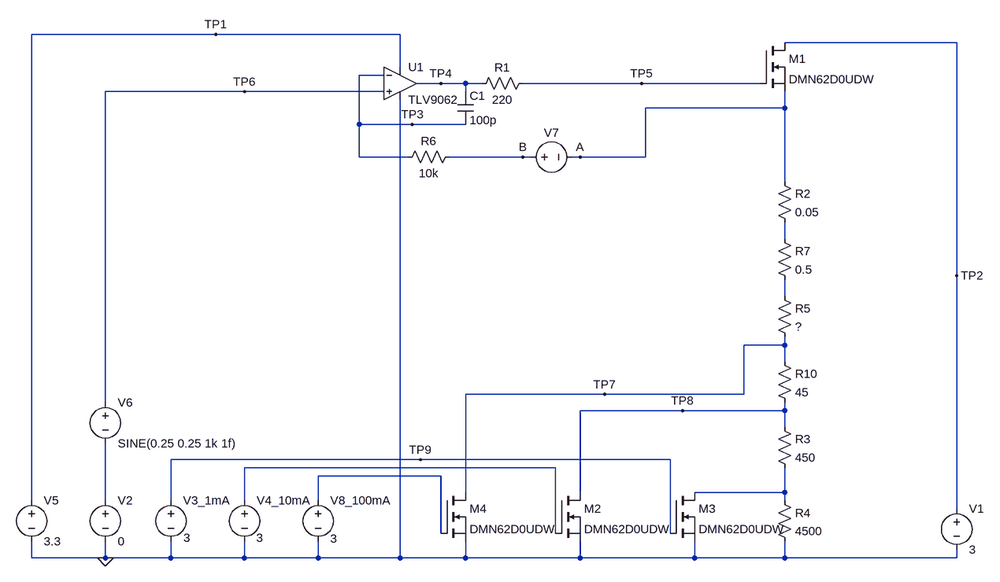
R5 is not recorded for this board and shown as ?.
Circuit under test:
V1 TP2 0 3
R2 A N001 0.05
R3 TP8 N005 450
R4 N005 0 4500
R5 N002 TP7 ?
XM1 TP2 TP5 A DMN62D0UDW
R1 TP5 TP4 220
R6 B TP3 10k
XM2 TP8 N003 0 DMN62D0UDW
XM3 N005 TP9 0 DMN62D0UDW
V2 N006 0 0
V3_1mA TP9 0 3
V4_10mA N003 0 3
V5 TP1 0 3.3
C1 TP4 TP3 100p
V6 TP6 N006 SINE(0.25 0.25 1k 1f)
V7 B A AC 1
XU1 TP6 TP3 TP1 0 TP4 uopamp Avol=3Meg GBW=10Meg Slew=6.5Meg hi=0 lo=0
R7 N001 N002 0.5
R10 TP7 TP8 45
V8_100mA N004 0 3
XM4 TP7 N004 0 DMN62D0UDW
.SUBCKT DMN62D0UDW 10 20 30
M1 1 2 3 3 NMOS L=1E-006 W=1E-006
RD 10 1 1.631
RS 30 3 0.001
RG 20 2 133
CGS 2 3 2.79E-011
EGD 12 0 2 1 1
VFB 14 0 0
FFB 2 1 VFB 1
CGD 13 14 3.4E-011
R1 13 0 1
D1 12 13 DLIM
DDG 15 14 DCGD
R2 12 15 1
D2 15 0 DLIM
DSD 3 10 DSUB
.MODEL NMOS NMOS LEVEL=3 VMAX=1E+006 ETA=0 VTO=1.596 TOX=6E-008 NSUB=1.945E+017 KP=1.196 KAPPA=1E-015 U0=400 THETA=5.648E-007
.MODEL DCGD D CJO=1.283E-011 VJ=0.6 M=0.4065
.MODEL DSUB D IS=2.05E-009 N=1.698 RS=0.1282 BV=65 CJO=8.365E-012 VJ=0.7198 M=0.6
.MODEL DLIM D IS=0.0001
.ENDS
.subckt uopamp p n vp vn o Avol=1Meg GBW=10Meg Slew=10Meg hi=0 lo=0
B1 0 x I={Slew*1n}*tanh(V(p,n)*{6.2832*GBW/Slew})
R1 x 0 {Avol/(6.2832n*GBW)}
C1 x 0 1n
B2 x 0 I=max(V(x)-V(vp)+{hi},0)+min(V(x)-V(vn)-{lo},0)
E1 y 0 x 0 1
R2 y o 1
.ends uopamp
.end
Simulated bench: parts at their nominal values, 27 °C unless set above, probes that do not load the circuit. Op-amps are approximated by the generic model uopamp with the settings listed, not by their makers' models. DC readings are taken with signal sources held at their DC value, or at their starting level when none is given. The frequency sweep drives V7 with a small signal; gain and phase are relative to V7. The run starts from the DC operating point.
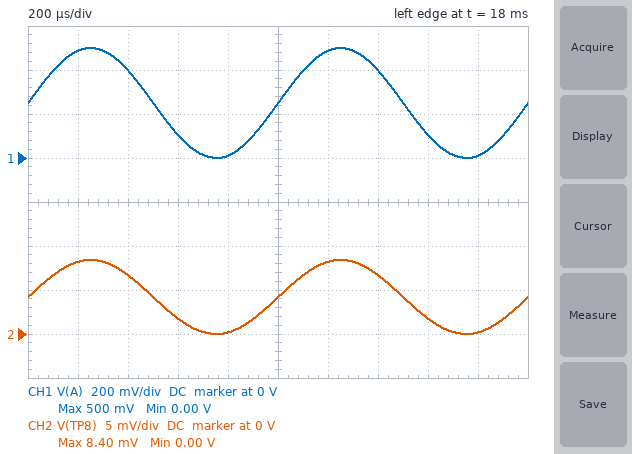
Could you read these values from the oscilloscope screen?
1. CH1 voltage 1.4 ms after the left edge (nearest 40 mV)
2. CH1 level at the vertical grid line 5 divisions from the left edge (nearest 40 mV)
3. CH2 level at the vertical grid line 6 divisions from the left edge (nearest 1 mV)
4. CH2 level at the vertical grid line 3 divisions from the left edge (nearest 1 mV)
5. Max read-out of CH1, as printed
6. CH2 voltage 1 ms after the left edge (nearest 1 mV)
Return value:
400 mV
240 mV
8 mV
2 mV
500 mV
4 mV
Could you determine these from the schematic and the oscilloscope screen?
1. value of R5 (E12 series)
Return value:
3.3 Ω
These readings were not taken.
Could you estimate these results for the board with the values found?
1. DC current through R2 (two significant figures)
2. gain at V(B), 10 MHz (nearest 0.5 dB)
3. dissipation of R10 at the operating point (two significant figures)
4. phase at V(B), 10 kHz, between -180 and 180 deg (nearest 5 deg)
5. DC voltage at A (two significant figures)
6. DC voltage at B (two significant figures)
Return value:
42 mA
0 dB
160 µW
85 deg
250 mV
250 mV
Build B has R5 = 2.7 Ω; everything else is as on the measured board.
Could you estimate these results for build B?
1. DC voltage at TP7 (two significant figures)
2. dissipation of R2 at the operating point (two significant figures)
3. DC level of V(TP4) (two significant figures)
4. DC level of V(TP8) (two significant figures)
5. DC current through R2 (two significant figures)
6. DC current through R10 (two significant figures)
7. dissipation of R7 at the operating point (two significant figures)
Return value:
99 mV
110 µW
2.3 V
4.7 mV
46 mA
2.1 mA
1.1 mW
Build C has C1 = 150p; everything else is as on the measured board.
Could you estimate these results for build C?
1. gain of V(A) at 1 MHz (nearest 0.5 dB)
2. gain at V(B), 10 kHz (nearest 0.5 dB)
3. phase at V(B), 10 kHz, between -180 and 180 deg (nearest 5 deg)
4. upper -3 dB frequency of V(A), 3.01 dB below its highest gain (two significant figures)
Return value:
-24.5 dB
-15.5 dB
80 deg
59 kHz
